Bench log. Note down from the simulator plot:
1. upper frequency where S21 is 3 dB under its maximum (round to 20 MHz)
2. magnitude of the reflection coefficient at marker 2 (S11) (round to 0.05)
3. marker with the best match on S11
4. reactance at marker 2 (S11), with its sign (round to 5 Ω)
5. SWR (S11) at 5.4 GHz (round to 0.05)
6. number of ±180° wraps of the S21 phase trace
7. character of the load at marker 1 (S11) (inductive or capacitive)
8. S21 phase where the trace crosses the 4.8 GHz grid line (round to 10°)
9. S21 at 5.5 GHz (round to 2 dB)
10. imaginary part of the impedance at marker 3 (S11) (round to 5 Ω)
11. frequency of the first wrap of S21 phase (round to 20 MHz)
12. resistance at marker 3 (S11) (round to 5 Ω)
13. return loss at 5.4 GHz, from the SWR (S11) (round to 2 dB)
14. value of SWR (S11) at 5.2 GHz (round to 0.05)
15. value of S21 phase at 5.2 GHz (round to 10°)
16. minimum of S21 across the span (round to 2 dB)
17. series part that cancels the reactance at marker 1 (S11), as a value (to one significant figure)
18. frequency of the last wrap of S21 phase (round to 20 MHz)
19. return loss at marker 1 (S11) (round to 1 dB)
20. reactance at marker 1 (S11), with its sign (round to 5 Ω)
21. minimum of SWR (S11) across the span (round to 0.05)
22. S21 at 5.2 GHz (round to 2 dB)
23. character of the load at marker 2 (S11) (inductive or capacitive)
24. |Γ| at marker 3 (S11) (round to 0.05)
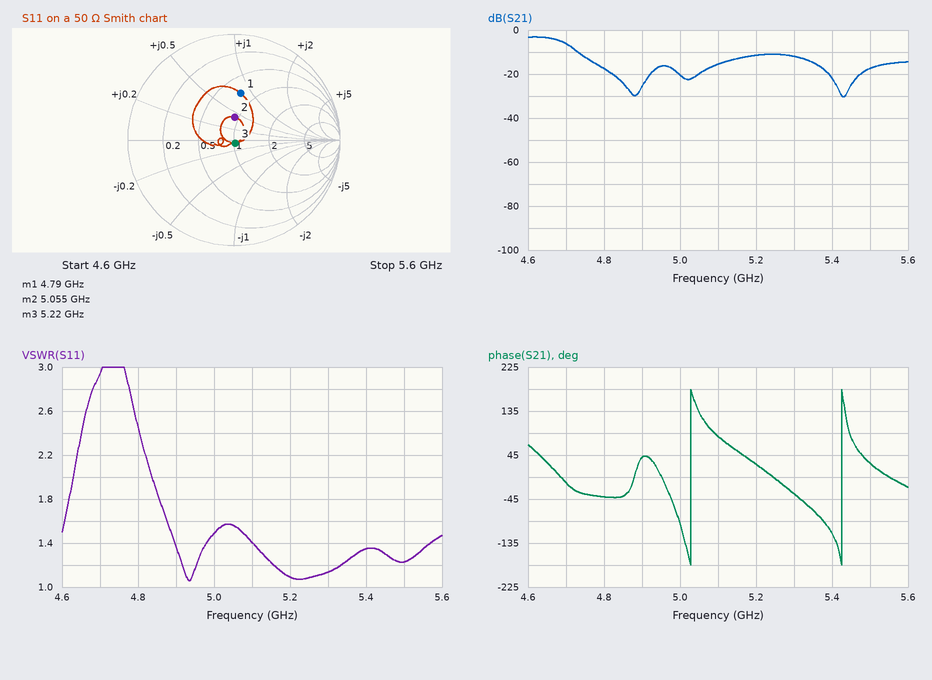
4.70 GHz
0.20
marker 3
+20 Ω
1.35
2
inductive
-40°
-18 dB
-5 Ω
5.02 GHz
50 Ω
16 dB
1.10
30°
-30 dB
800 fF
5.42 GHz
7 dB
+40 Ω
1.05
-12 dB
inductive
0.05
